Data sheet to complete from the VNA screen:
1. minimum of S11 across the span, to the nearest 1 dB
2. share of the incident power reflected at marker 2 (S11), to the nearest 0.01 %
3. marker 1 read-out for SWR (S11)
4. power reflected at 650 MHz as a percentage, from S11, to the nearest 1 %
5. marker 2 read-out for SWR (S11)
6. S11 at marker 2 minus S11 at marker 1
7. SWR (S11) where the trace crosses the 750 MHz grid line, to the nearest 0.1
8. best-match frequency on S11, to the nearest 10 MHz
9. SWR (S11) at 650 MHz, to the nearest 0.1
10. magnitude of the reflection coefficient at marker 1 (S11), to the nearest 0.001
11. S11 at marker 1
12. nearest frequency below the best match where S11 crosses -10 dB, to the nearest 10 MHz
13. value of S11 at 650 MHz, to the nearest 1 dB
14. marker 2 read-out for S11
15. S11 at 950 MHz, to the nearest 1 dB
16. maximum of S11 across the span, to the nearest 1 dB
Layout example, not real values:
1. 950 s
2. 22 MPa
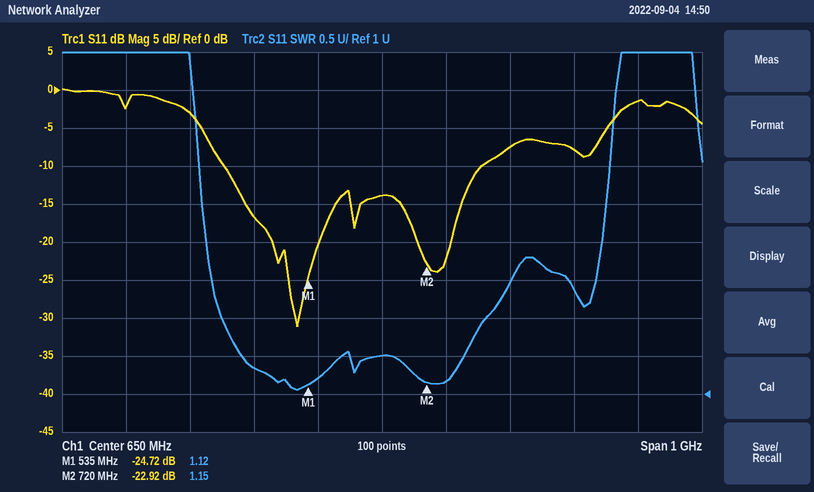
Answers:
1. -31 dB
2. 0.51 %
3. 1.12
4. 4 %
5. 1.15
6. 1.80 dB
7. 1.2
8. 520 MHz
9. 1.5
10. 0.058
11. -24.72 dB
12. 400 MHz
13. -14 dB
14. -22.92 dB
15. -8 dB
16. 0 dB
